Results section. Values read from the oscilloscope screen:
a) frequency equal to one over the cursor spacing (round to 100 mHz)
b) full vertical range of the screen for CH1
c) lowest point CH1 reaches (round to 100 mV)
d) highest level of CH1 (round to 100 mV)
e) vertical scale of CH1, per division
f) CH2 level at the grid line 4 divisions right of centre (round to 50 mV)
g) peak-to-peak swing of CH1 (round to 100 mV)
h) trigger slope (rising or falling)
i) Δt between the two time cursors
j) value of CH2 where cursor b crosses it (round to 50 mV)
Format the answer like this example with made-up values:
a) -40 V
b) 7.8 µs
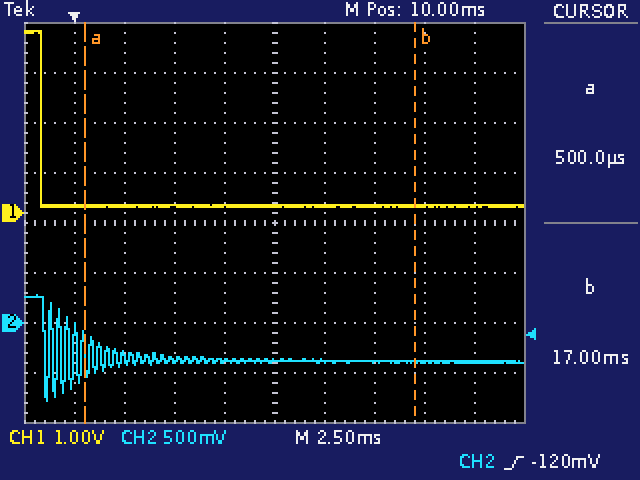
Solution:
a) 60.6 Hz
b) 8 V
c) 100 mV
d) 3.6 V
e) 1 V
f) -400 mV
g) 3.5 V
h) rising
i) 16.50 ms
j) -400 mV
